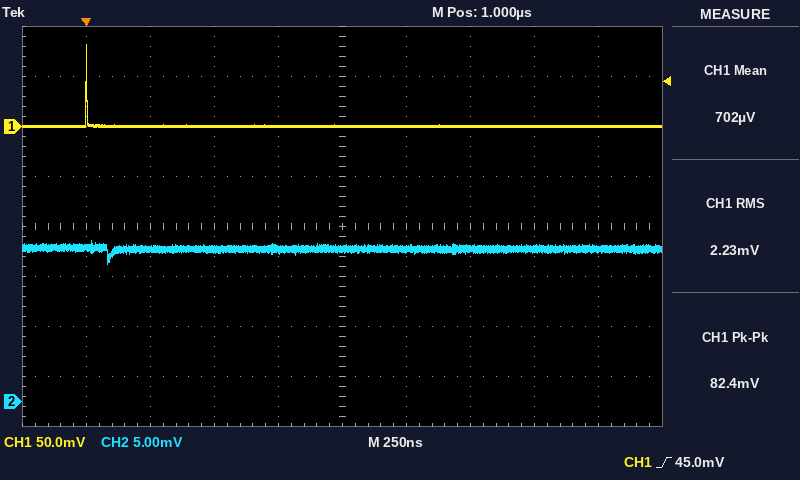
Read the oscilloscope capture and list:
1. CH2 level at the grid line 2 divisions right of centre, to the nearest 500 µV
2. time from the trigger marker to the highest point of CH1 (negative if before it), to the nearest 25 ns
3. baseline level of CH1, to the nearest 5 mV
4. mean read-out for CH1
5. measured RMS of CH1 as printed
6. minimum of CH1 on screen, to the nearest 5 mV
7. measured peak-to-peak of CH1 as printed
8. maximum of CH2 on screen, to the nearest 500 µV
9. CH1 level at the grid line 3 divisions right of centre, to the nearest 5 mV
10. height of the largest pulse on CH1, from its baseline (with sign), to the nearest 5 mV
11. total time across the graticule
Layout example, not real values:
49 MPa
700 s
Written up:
15.5 mV
0 ns
0 mV
702 µV
2.23 mV
0 mV
82.4 mV
16.0 mV
0 mV
+80 mV
2.5 µs
